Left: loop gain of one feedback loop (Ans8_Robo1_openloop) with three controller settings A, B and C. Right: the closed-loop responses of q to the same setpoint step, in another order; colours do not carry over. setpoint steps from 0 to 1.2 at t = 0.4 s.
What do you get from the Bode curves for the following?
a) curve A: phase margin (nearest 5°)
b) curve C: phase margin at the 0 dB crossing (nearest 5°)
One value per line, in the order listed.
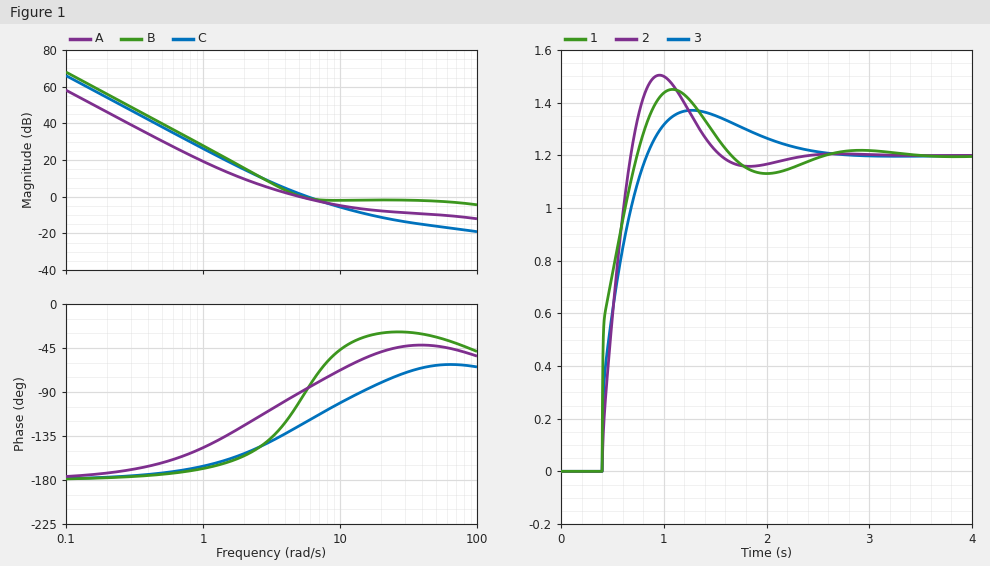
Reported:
90°
60°
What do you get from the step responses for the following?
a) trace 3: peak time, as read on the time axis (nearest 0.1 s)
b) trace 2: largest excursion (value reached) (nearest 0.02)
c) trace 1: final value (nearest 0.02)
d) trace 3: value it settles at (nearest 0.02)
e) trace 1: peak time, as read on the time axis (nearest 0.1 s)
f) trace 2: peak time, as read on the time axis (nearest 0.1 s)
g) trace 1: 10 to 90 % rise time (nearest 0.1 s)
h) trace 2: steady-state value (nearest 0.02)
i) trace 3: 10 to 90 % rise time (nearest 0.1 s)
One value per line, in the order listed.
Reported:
1.3 s
1.50
1.20
1.20
1.1 s
1.0 s
0.3 s
1.20
0.3 s
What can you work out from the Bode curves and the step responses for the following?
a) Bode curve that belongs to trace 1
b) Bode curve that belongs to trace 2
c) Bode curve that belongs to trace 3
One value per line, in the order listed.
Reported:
B
C
A
